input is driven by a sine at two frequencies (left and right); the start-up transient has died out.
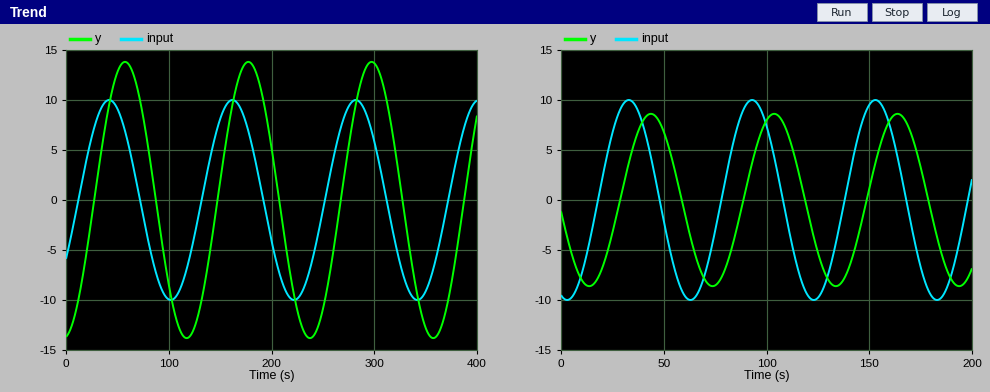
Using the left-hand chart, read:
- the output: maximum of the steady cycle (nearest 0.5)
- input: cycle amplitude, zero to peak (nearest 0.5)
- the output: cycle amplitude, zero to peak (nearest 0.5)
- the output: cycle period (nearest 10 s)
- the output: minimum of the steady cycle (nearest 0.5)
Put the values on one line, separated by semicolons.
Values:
14.0; 10.0; 14.0; 120 s; -14.0
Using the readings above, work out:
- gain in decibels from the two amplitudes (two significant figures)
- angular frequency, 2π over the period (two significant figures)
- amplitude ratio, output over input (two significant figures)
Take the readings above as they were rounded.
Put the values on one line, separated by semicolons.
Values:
2.9 dB; 0.052 rad/s; 1.4
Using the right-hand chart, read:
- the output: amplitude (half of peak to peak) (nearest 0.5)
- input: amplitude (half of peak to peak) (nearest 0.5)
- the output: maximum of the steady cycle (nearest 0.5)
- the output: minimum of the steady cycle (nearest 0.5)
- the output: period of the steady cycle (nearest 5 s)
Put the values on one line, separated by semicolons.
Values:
8.5; 10.0; 8.5; -8.5; 60 s
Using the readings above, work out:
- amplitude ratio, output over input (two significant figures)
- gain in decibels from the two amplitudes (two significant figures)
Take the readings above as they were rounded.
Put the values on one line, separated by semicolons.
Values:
0.85; -1.4 dB
